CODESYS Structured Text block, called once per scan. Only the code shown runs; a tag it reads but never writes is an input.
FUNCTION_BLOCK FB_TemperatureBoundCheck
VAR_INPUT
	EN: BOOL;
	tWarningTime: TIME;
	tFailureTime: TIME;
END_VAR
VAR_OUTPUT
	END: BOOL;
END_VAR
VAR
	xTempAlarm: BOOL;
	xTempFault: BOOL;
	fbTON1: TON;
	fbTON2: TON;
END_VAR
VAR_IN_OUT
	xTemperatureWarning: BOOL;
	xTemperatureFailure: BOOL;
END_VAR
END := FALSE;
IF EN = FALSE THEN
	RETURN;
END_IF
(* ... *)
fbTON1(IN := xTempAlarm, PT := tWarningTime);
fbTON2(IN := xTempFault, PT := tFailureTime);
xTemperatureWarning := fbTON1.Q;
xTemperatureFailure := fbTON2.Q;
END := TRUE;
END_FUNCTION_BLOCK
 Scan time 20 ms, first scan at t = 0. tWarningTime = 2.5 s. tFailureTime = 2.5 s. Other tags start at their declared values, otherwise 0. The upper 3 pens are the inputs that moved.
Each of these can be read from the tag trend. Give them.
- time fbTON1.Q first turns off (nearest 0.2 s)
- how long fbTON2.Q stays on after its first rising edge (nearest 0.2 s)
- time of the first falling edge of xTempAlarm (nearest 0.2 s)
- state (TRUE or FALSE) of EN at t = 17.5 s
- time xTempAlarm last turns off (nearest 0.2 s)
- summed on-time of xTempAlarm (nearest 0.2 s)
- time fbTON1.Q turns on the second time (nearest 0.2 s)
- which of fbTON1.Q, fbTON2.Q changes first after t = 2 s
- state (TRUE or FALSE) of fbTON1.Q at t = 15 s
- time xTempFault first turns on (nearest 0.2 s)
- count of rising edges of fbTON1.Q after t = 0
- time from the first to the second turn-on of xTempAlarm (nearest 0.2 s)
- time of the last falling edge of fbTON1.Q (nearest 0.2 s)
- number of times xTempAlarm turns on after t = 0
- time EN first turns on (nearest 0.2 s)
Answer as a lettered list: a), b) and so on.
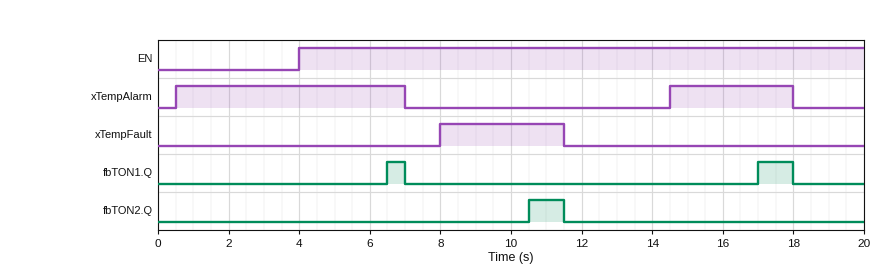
a) 7.0 s
b) 1.0 s
c) 7.0 s
d) TRUE
e) 18.0 s
f) 10.0 s
g) 17.0 s
h) fbTON1.Q
i) FALSE
j) 8.0 s
k) 2
l) 14.0 s
m) 18.0 s
n) 2
o) 4.0 s
